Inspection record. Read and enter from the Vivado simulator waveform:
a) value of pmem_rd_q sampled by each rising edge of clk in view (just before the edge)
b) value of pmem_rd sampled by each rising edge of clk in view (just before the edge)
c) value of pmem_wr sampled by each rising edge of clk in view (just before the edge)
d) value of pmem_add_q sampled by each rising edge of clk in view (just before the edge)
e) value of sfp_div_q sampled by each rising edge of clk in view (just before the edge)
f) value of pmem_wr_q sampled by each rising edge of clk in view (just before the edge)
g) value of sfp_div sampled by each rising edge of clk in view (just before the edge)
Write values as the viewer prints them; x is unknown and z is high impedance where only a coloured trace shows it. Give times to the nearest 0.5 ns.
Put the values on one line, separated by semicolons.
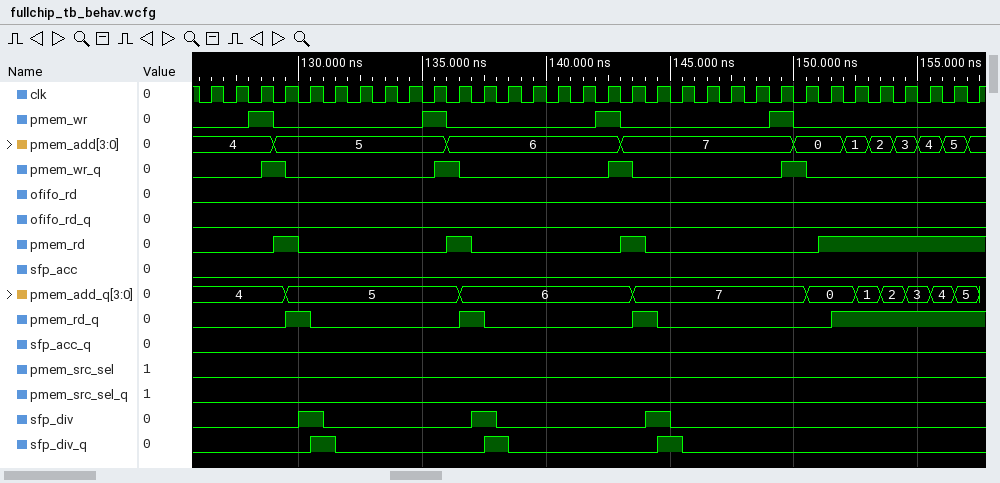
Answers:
0 0 0 0 1 0 0 0 0 0 0 1 0 0 0 0 0 0 1 0 0 0 0 0 0 0 1 1 1 1 1 1; 0 0 0 1 0 0 0 0 0 0 1 0 0 0 0 0 0 1 0 0 0 0 0 0 0 1 1 1 1 1 1 1; 0 0 1 0 0 0 0 0 0 1 0 0 0 0 0 0 1 0 0 0 0 0 0 1 0 0 0 0 0 0 0 0; 4, 4, 4, 4, 5, 5, 5, 5, 5, 5, 5, 6, 6, 6, 6, 6, 6, 6, 7, 7, 7, 7, 7, 7, 7, 0, 0, 1, 2, 3, 4, 5; 0 0 0 0 0 1 0 0 0 0 0 0 1 0 0 0 0 0 0 1 0 0 0 0 0 0 0 0 0 0 0 0; 0 0 0 1 0 0 0 0 0 0 1 0 0 0 0 0 0 1 0 0 0 0 0 0 1 0 0 0 0 0 0 0; 0 0 0 0 1 0 0 0 0 0 0 1 0 0 0 0 0 0 1 0 0 0 0 0 0 0 0 0 0 0 0 0
